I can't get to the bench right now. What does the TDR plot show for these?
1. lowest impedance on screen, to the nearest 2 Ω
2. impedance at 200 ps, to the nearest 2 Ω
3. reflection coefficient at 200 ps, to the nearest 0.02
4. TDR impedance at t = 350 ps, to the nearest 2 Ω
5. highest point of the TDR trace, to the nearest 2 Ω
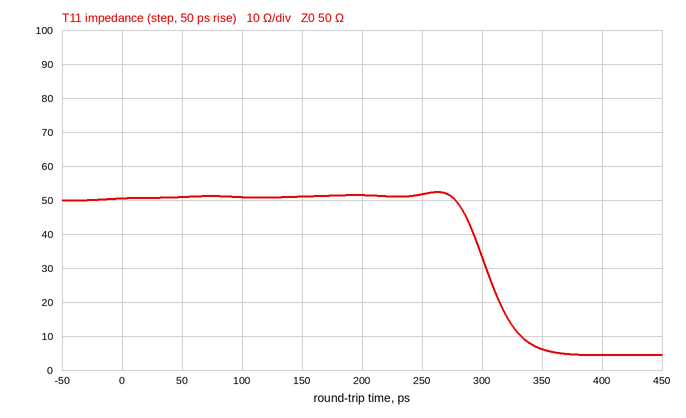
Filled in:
4 Ω
52 Ω
+0.02
6 Ω
52 Ω
